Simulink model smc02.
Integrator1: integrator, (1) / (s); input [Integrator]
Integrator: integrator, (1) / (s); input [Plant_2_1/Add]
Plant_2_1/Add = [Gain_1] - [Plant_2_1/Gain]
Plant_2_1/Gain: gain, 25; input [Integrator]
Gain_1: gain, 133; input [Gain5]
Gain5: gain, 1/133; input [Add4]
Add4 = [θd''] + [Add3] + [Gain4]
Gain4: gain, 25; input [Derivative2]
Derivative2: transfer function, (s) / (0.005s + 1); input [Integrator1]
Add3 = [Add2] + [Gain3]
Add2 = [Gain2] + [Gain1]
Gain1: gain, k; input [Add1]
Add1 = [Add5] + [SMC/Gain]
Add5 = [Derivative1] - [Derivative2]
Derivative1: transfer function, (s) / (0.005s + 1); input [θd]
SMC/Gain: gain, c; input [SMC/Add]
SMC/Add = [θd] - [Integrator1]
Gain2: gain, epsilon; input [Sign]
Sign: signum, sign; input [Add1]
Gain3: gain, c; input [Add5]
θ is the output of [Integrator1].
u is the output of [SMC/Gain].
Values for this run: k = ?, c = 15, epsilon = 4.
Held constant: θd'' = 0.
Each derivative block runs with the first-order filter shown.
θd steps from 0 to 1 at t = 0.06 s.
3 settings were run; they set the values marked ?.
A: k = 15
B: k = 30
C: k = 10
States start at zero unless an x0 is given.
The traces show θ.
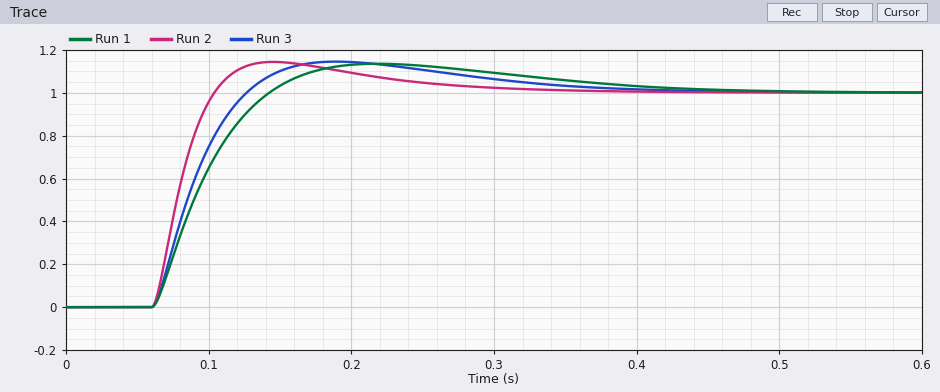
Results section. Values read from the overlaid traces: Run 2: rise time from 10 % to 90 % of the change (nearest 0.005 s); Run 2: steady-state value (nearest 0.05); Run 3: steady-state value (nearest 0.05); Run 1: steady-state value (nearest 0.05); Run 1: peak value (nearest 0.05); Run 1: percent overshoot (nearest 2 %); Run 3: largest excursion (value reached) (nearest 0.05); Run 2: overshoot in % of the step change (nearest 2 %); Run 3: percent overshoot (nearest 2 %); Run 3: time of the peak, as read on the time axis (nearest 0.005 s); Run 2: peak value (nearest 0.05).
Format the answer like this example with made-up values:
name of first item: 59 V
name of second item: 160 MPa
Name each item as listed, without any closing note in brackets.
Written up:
Run 2: rise time from 10 % to 90 % of the change: 0.030 s
Run 2: steady-state value: 1.00
Run 3: steady-state value: 1.00
Run 1: steady-state value: 1.00
Run 1: peak value: 1.15
Run 1: percent overshoot: 14 %
Run 3: largest excursion (value reached): 1.15
Run 2: overshoot in % of the step change: 14 %
Run 3: percent overshoot: 14 %
Run 3: time of the peak, as read on the time axis: 0.190 s
Run 2: peak value: 1.15
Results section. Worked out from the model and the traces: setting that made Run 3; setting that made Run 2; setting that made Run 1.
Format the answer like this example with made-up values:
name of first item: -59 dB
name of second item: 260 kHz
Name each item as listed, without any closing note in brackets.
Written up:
setting that made Run 3: A
setting that made Run 2: B
setting that made Run 1: C
